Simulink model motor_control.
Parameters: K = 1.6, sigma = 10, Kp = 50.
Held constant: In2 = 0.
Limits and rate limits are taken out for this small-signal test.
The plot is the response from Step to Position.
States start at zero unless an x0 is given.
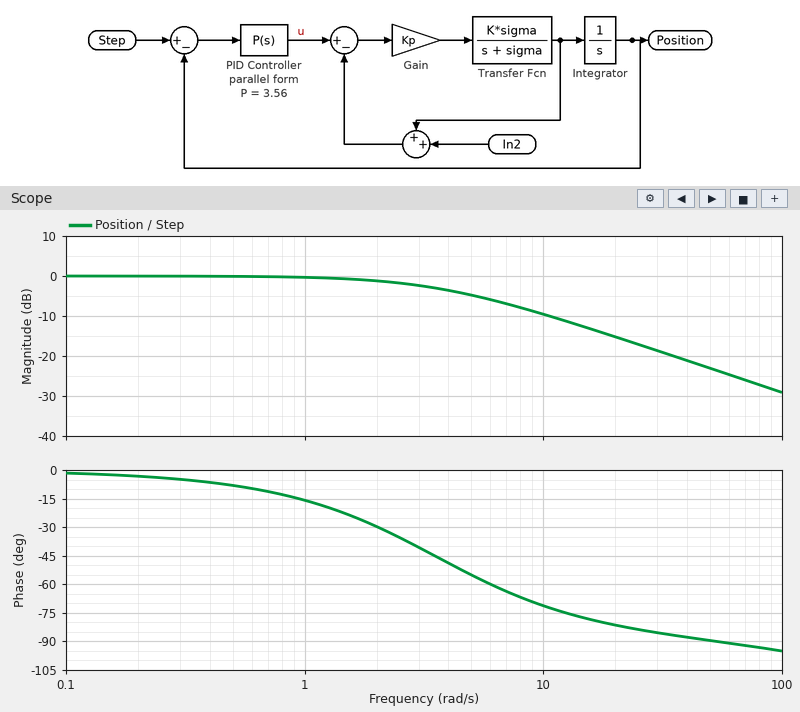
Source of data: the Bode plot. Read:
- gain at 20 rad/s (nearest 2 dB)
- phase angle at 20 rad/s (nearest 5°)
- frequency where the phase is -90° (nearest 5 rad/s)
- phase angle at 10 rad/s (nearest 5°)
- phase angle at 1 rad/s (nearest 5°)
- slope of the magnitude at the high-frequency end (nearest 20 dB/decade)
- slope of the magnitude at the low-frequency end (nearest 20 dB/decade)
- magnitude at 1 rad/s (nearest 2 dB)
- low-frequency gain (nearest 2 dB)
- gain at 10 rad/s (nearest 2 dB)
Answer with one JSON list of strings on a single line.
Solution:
["-16 dB", "-80°", "55 rad/s", "-70°", "-15°", "-20 dB/decade", "0 dB/decade", "0 dB", "0 dB", "-10 dB"]
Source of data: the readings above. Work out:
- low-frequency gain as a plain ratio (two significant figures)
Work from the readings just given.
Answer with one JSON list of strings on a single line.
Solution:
["1.0"]
